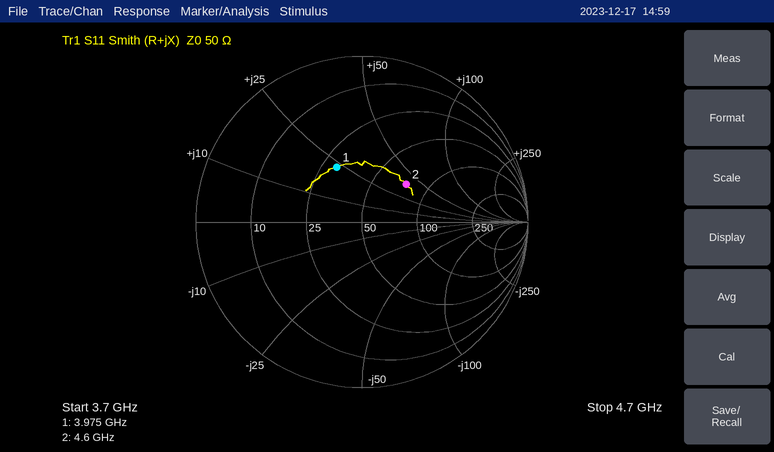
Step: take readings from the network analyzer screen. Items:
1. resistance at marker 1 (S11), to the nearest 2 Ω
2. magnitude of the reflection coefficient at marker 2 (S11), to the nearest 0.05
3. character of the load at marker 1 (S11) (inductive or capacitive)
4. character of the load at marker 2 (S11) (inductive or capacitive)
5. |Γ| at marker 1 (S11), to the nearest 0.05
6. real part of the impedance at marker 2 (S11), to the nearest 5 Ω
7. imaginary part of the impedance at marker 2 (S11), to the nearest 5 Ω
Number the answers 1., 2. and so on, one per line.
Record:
1. 30 Ω
2. 0.35
3. inductive
4. inductive
5. 0.35
6. 75 Ω
7. +40 Ω
